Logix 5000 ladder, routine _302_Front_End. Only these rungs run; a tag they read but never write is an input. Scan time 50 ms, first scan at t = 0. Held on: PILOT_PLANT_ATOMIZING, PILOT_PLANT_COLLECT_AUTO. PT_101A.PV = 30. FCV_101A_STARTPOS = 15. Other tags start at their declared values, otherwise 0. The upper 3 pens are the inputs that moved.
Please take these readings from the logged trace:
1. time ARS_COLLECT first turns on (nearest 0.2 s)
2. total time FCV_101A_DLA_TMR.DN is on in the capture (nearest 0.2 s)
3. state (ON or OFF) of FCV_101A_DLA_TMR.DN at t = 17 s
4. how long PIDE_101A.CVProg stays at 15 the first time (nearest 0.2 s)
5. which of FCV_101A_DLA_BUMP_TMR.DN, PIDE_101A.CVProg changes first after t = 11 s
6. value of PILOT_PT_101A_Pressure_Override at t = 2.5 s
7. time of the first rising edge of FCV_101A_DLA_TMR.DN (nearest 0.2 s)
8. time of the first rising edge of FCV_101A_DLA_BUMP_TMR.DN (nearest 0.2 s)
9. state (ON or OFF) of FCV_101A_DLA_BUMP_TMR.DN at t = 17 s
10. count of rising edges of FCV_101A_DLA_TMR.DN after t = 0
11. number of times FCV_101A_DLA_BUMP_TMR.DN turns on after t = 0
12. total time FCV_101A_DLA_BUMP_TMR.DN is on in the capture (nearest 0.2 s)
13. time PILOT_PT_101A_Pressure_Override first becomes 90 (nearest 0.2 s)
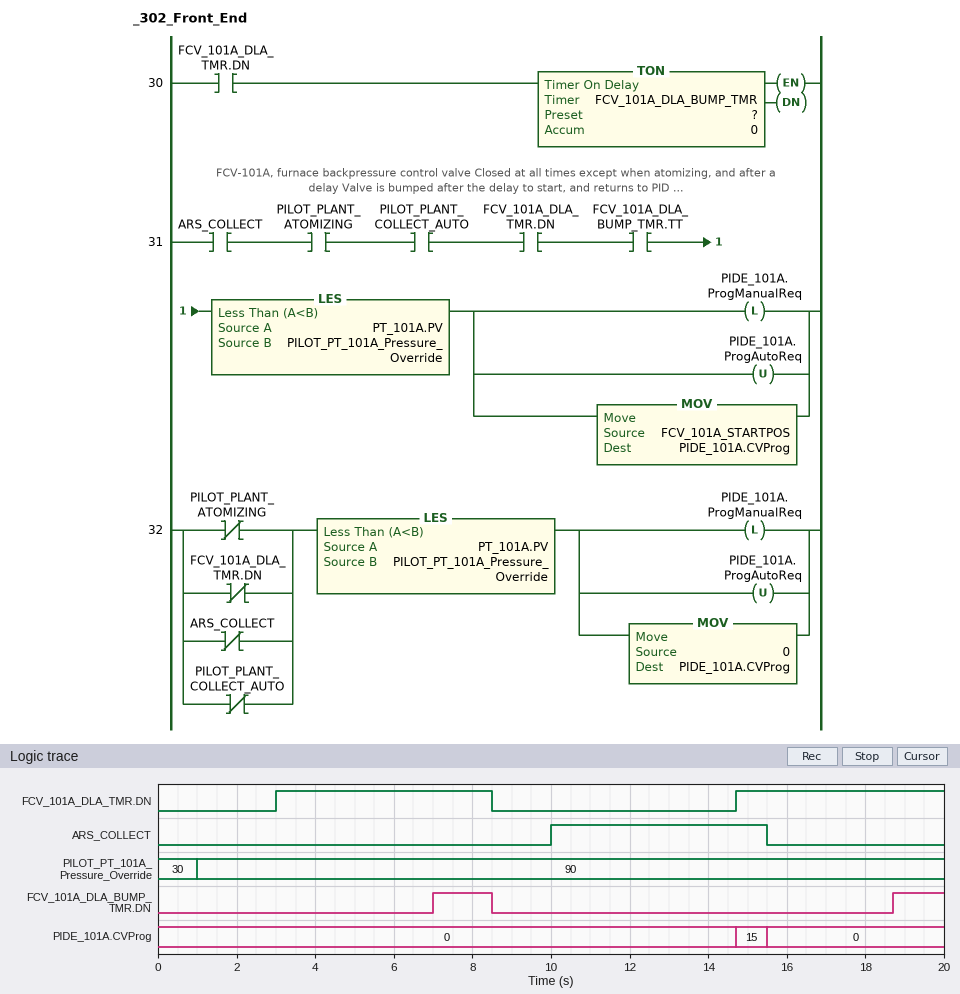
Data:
10.0 s
10.8 s
ON
0.8 s
PIDE_101A.CVProg
90
3.0 s
7.0 s
OFF
2
2
2.8 s
1.0 s
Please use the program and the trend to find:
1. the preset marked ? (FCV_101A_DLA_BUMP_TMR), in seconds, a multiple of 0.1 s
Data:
4.0 s
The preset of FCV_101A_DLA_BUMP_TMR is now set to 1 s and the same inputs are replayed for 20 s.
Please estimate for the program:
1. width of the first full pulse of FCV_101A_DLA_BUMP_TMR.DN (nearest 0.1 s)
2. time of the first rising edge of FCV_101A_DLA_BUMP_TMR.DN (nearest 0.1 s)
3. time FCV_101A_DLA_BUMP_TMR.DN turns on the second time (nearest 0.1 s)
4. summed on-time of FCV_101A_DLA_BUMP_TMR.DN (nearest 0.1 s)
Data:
4.5 s
4.0 s
15.7 s
8.8 s
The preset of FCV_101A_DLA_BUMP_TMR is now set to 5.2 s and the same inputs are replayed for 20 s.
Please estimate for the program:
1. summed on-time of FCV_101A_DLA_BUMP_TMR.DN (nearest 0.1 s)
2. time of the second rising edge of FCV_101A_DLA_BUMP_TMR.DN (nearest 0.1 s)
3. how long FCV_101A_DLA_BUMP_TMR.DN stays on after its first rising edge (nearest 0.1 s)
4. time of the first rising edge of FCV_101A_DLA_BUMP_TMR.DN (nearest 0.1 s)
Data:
0.4 s
19.9 s
0.3 s
8.2 s
